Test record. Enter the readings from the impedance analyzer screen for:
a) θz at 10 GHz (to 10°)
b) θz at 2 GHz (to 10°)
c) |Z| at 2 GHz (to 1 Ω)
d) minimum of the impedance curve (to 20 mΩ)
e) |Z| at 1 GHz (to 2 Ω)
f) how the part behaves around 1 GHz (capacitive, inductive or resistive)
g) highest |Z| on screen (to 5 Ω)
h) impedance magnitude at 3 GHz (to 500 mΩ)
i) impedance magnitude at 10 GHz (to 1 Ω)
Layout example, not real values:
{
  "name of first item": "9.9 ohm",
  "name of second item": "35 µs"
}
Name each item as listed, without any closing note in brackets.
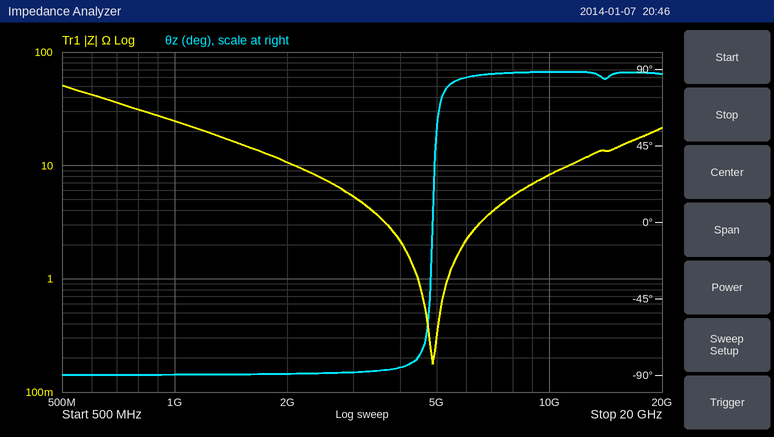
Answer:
{
  "θz at 10 GHz": "90°",
  "θz at 2 GHz": "-90°",
  "|Z| at 2 GHz": "11 Ω",
  "minimum of the impedance curve": "180 mΩ",
  "|Z| at 1 GHz": "24 Ω",
  "how the part behaves around 1 GHz": "capacitive",
  "highest |Z| on screen": "50 Ω",
  "impedance magnitude at 3 GHz": "5.5 Ω",
  "impedance magnitude at 10 GHz": "8 Ω"
}
